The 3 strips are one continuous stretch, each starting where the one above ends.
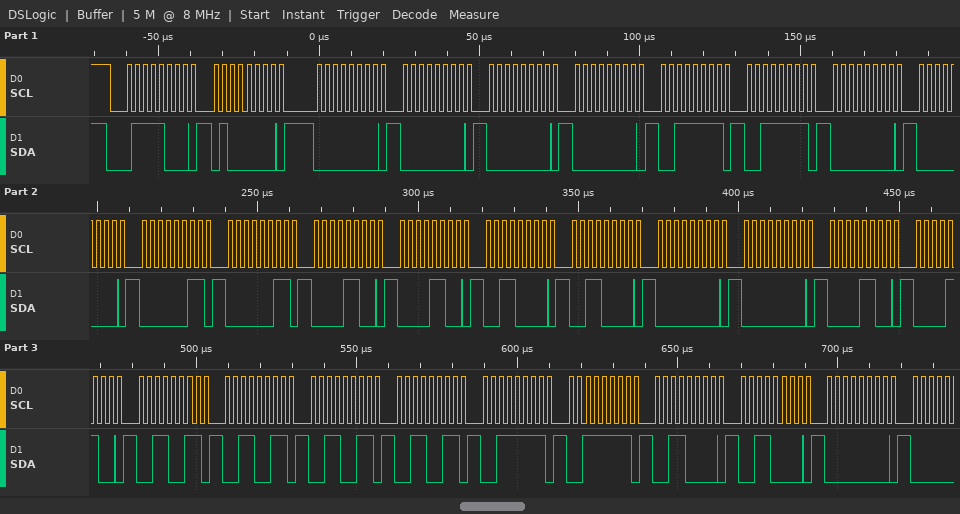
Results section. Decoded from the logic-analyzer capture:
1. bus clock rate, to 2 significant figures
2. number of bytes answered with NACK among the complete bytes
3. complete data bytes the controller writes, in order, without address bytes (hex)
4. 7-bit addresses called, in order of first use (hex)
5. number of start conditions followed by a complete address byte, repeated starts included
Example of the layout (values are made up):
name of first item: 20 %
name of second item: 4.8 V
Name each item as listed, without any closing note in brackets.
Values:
bus clock rate, to 2 significant figures: 400 kHz
number of bytes answered with NACK among the complete bytes: 0
complete data bytes the controller writes, in order, without address bytes: 40 00 00 00 00 3F 3F 00 00 03 03 0C 0C 30 30 00 00 0C 0C 33 33 33 33 3F 3F 30 30 00
7-bit addresses called, in order of first use: 0x3C
number of start conditions followed by a complete address byte, repeated starts included: 1
